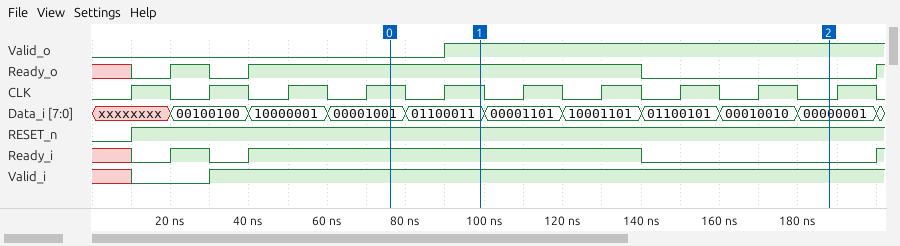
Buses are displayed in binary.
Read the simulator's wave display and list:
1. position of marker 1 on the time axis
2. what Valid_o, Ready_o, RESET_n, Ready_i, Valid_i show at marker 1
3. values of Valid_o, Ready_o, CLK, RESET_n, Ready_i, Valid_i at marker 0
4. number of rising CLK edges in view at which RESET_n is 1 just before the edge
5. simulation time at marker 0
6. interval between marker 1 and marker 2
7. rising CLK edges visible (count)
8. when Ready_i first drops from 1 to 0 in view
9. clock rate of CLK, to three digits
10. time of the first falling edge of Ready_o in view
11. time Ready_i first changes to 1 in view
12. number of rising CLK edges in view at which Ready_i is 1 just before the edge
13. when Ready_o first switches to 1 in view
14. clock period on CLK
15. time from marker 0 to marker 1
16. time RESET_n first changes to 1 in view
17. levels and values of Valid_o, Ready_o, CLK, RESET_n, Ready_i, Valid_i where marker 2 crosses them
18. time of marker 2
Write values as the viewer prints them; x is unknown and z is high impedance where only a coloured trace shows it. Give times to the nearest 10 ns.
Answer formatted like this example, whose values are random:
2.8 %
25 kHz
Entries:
100 ns
Valid_o=1, Ready_o=1, RESET_n=1, Ready_i=1, Valid_i=1
Valid_o=0, Ready_o=1, CLK=1, RESET_n=1, Ready_i=1, Valid_i=1
9
80 ns
90 ns
10
30 ns
50.0 MHz
30 ns
20 ns
6
20 ns
20 ns
20 ns
10 ns
Valid_o=1, Ready_o=0, CLK=0, RESET_n=1, Ready_i=0, Valid_i=1
190 ns
